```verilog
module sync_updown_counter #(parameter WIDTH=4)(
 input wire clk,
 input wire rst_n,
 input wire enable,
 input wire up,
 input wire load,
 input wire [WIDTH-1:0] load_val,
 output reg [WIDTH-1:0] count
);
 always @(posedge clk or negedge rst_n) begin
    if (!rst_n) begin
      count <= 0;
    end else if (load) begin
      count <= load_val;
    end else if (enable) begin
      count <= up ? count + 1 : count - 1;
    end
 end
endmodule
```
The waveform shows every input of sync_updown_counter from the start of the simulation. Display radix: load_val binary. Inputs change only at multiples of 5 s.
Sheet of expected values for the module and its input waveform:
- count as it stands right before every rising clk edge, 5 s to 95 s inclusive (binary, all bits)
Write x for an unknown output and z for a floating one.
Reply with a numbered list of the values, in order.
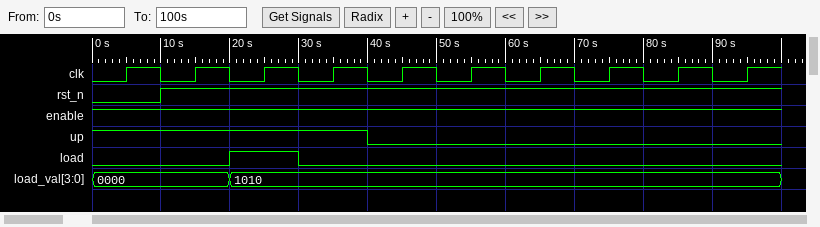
1. 0000, 0000, 0001, 1010, 1011, 1010, 1001, 1000, 0111, 0110
